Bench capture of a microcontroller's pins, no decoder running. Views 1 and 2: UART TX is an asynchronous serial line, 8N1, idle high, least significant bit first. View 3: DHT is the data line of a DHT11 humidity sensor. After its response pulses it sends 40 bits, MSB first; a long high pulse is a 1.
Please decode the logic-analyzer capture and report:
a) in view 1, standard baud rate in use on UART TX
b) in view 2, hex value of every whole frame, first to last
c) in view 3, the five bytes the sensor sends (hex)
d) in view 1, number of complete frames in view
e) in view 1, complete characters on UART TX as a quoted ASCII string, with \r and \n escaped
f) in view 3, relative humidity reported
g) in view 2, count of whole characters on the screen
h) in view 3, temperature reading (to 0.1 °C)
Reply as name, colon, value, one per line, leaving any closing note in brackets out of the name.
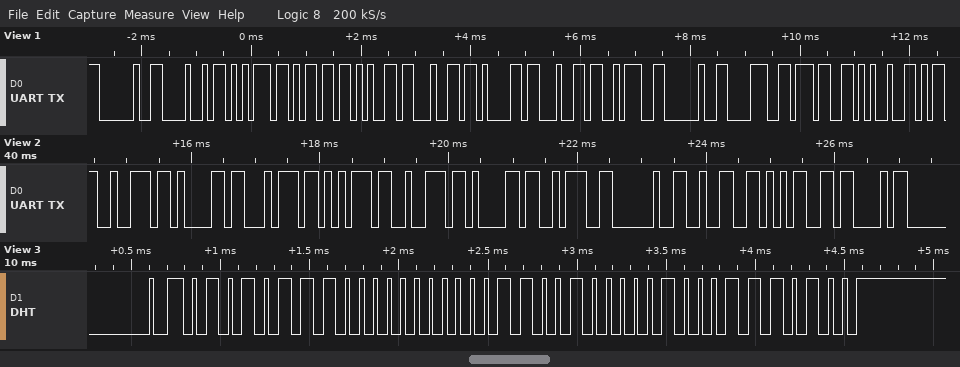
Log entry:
in view 1, standard baud rate in use on UART TX: 9600 baud
in view 2, hex value of every whole frame, first to last: 72 61 74 75 72 61 3A 20 32 35 43
in view 3, the five bytes the sensor sends: 57 00 19 04 74
in view 1, number of complete frames in view: 13
in view 1, complete characters on UART TX as a quoted ASCII string, with \r and \n escaped: " Humedad: 87%"
in view 3, relative humidity reported: 87 %
in view 2, count of whole characters on the screen: 11
in view 3, temperature reading: 25.4 °C
